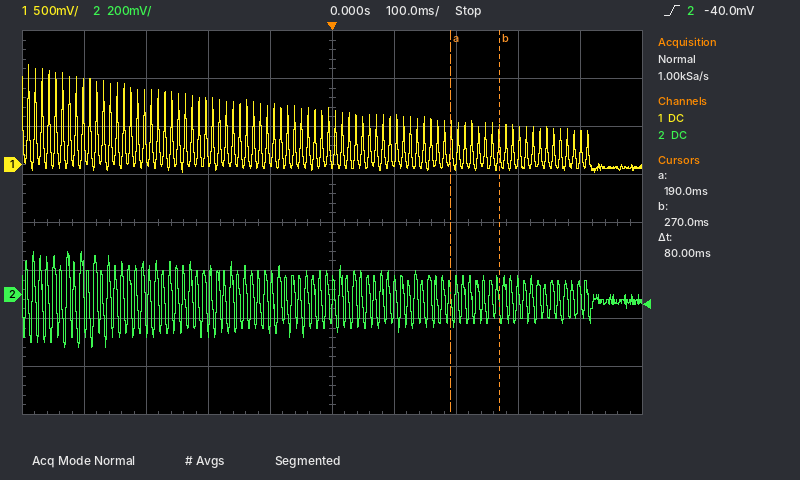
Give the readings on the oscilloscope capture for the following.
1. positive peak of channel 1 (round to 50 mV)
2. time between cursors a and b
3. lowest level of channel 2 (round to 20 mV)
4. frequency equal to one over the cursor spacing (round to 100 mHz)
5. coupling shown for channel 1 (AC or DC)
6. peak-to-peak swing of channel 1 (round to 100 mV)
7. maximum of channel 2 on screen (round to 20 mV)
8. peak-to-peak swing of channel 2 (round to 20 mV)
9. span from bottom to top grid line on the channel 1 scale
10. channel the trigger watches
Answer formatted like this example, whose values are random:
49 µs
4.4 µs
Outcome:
1.05 V
80 ms
-220 mV
12.5 Hz
DC
1.10 V
180 mV
400 mV
4 V
channel 2
